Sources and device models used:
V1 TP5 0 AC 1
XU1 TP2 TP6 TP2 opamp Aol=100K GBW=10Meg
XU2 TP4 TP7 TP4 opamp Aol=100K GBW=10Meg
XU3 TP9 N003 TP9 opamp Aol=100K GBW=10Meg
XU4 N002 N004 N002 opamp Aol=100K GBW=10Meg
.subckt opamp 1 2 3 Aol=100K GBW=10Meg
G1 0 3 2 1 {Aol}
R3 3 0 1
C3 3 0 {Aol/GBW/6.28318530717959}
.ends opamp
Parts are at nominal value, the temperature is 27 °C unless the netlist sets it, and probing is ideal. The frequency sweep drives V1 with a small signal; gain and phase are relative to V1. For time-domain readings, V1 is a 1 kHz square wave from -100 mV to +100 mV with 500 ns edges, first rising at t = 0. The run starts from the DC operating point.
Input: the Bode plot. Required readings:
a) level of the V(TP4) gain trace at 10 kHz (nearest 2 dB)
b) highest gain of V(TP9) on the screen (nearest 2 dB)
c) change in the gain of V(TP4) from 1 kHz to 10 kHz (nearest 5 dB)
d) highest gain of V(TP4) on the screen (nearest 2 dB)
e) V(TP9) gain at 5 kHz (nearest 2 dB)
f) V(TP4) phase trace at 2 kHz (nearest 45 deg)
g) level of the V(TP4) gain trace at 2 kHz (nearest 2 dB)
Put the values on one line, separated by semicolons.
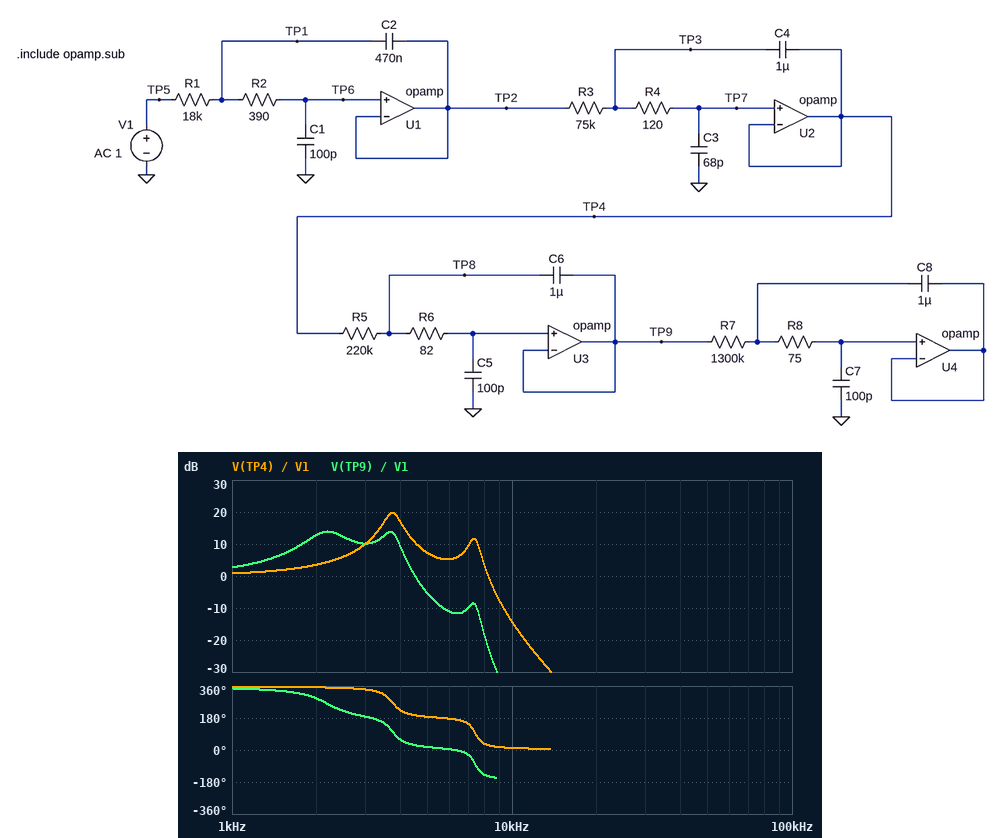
-14 dB; 14 dB; -15 dB; 20 dB; -6 dB; 360 deg; 4 dB
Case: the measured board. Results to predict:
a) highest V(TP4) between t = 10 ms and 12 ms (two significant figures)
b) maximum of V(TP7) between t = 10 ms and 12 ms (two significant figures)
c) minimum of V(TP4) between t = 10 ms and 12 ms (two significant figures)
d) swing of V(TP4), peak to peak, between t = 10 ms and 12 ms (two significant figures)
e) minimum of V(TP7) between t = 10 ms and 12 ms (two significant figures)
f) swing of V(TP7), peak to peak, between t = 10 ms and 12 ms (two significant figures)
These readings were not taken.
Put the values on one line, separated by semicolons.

320 mV; 320 mV; -320 mV; 640 mV; -320 mV; 640 mV
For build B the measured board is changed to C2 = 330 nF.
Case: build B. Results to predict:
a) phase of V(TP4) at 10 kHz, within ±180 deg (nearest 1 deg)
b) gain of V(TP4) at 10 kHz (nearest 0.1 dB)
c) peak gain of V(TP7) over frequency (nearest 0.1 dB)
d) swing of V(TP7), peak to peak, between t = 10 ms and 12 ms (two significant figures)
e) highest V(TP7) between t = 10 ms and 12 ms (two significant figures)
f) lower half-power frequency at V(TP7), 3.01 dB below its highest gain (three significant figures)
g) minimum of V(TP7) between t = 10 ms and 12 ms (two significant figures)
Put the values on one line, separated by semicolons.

26 deg; -5.6 dB; 18.9 dB; 570 mV; 290 mV; 3.47 kHz; -290 mV
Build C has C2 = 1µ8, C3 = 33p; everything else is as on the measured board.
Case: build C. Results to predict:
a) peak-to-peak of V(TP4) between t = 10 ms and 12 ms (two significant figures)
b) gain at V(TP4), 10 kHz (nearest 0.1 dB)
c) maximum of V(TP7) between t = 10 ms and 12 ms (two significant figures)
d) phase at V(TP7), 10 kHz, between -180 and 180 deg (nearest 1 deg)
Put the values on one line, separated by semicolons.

750 mV; -29.4 dB; 370 mV; 4 deg
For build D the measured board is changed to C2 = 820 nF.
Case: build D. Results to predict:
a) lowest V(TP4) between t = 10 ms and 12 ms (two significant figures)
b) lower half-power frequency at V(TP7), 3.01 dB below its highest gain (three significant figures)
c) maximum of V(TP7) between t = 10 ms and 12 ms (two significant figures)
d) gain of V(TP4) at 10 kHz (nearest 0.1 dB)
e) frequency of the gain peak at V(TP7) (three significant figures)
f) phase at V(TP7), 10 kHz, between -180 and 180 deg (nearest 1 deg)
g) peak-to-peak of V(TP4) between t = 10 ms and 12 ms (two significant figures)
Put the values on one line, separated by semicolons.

-370 mV; 3.51 kHz; 370 mV; -22.6 dB; 3.76 kHz; 7 deg; 740 mV
